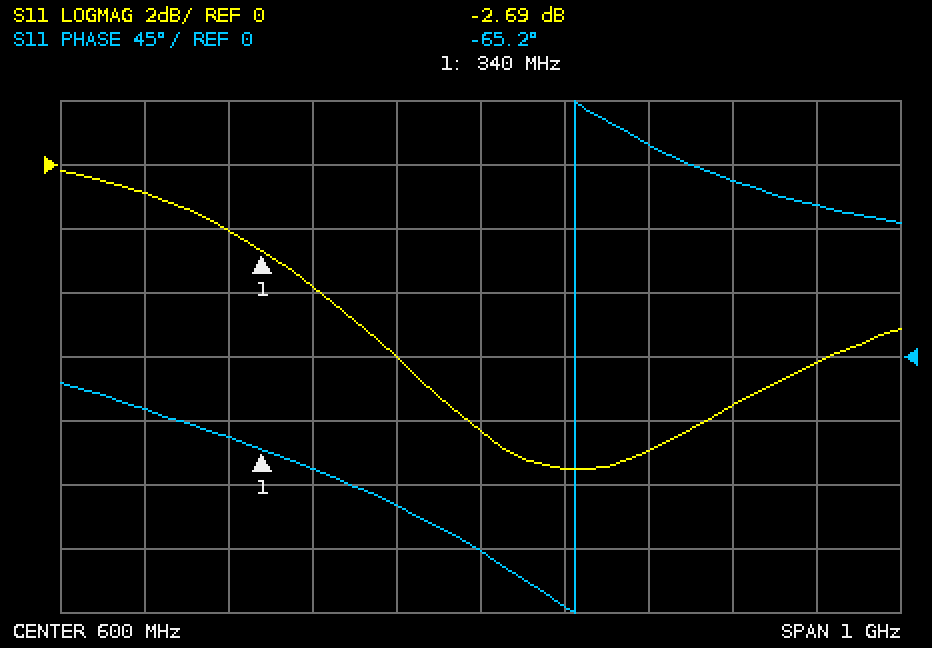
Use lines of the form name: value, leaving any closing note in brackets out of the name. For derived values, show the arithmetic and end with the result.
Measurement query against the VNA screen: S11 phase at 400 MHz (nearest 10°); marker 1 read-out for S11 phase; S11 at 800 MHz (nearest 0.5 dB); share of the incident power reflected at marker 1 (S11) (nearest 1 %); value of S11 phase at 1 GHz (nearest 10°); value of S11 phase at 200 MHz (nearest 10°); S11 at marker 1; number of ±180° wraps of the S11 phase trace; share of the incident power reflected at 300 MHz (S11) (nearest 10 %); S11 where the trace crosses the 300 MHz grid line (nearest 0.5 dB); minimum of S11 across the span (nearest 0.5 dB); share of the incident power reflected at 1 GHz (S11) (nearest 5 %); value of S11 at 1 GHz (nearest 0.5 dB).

S11 phase at 400 MHz: -80°
marker 1 read-out for S11 phase: -65.2°
S11 at 800 MHz: -9.0 dB
share of the incident power reflected at marker 1 (S11): 10^(-2.69/10) ≈ 54 %
value of S11 phase at 1 GHz: 110°
value of S11 phase at 200 MHz: -40°
S11 at marker 1: -2.69 dB
number of ±180° wraps of the S11 phase trace: 1
share of the incident power reflected at 300 MHz (S11): 10^(-2/10) ≈ 63.1 %, so 60 % to the nearest 10 %
S11 where the trace crosses the 300 MHz grid line: -2.0 dB
minimum of S11 across the span: -9.5 dB
share of the incident power reflected at 1 GHz (S11): 10^(-6/10) ≈ 25 %
value of S11 at 1 GHz: -6.0 dB
